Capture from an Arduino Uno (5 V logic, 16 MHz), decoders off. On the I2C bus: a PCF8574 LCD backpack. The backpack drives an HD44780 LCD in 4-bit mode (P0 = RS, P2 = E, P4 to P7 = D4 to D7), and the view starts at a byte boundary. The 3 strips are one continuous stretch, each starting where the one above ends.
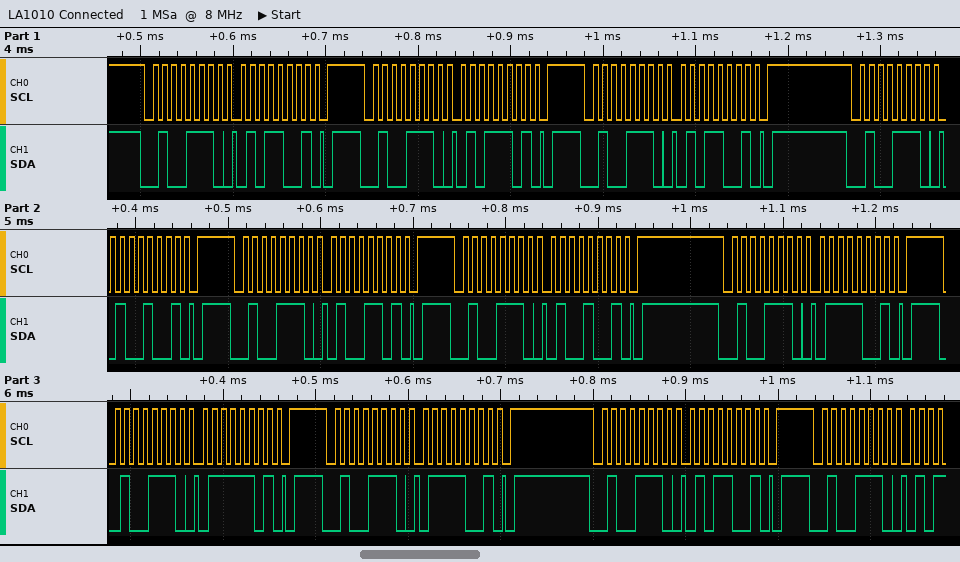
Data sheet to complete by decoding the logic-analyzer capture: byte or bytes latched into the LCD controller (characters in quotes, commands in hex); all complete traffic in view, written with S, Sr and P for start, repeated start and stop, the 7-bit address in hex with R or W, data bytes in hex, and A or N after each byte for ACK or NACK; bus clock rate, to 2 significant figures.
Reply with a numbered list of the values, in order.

1. 'T'
2. S 27W A 59 A P S 27W A 5D A P S 27W A 59 A P S 27W A 49 A P S 27W A 4D A P S 27W A 49 A P S 27W A 79 A P S 27W A 7D A P S 27W A 79 A P S 27W A 59 A P S 27W A
3. 100 kHz
